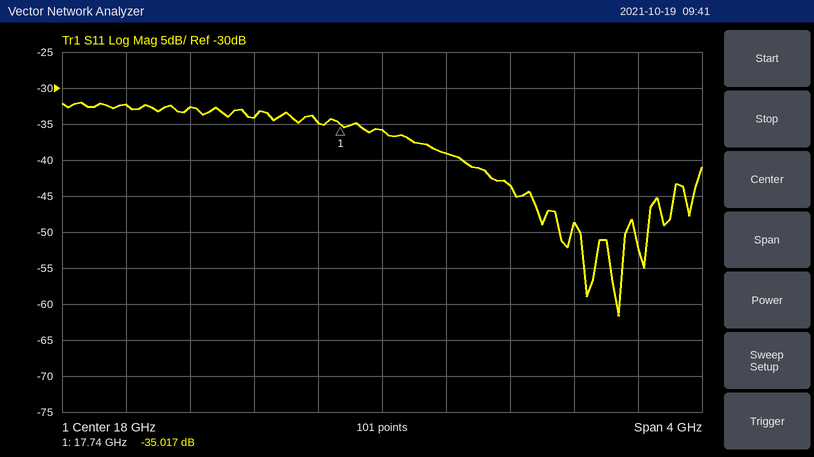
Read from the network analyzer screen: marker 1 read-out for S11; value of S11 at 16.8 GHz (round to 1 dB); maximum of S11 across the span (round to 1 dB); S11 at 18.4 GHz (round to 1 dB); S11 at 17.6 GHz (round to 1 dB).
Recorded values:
-35.017 dB
-33 dB
-32 dB
-39 dB
-35 dB
